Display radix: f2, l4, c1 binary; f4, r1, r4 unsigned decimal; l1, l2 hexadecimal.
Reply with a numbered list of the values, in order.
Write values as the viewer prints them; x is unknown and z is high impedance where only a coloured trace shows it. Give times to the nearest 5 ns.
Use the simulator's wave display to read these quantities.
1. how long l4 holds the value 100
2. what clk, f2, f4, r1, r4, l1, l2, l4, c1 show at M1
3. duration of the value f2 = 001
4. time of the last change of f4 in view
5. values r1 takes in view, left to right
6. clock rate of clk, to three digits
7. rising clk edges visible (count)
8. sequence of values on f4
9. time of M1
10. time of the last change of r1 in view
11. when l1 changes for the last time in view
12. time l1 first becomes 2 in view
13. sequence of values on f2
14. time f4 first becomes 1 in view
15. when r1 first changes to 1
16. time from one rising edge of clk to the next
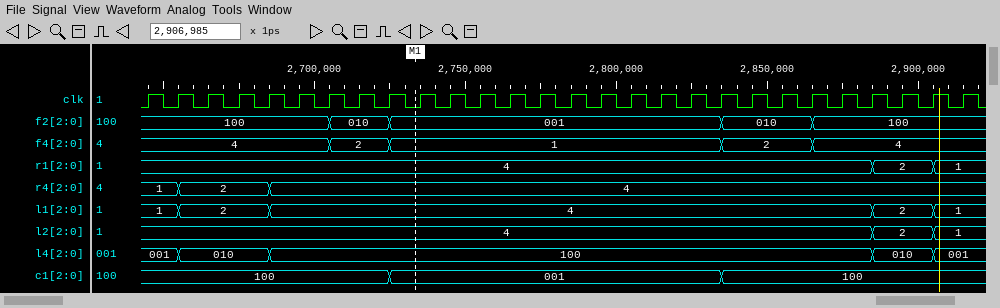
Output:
1. 200 ns
2. clk=0, f2=001, f4=1, r1=4, r4=4, l1=4, l2=4, l4=100, c1=001
3. 110 ns
4. 2865 ns
5. 4, 2, 1
6. 100 MHz
7. 28
8. 4, 2, 1, 2, 4
9. 2735 ns
10. 2905 ns
11. 2905 ns
12. 2655 ns
13. 100, 010, 001, 010, 100
14. 2725 ns
15. 2905 ns
16. 10 ns
